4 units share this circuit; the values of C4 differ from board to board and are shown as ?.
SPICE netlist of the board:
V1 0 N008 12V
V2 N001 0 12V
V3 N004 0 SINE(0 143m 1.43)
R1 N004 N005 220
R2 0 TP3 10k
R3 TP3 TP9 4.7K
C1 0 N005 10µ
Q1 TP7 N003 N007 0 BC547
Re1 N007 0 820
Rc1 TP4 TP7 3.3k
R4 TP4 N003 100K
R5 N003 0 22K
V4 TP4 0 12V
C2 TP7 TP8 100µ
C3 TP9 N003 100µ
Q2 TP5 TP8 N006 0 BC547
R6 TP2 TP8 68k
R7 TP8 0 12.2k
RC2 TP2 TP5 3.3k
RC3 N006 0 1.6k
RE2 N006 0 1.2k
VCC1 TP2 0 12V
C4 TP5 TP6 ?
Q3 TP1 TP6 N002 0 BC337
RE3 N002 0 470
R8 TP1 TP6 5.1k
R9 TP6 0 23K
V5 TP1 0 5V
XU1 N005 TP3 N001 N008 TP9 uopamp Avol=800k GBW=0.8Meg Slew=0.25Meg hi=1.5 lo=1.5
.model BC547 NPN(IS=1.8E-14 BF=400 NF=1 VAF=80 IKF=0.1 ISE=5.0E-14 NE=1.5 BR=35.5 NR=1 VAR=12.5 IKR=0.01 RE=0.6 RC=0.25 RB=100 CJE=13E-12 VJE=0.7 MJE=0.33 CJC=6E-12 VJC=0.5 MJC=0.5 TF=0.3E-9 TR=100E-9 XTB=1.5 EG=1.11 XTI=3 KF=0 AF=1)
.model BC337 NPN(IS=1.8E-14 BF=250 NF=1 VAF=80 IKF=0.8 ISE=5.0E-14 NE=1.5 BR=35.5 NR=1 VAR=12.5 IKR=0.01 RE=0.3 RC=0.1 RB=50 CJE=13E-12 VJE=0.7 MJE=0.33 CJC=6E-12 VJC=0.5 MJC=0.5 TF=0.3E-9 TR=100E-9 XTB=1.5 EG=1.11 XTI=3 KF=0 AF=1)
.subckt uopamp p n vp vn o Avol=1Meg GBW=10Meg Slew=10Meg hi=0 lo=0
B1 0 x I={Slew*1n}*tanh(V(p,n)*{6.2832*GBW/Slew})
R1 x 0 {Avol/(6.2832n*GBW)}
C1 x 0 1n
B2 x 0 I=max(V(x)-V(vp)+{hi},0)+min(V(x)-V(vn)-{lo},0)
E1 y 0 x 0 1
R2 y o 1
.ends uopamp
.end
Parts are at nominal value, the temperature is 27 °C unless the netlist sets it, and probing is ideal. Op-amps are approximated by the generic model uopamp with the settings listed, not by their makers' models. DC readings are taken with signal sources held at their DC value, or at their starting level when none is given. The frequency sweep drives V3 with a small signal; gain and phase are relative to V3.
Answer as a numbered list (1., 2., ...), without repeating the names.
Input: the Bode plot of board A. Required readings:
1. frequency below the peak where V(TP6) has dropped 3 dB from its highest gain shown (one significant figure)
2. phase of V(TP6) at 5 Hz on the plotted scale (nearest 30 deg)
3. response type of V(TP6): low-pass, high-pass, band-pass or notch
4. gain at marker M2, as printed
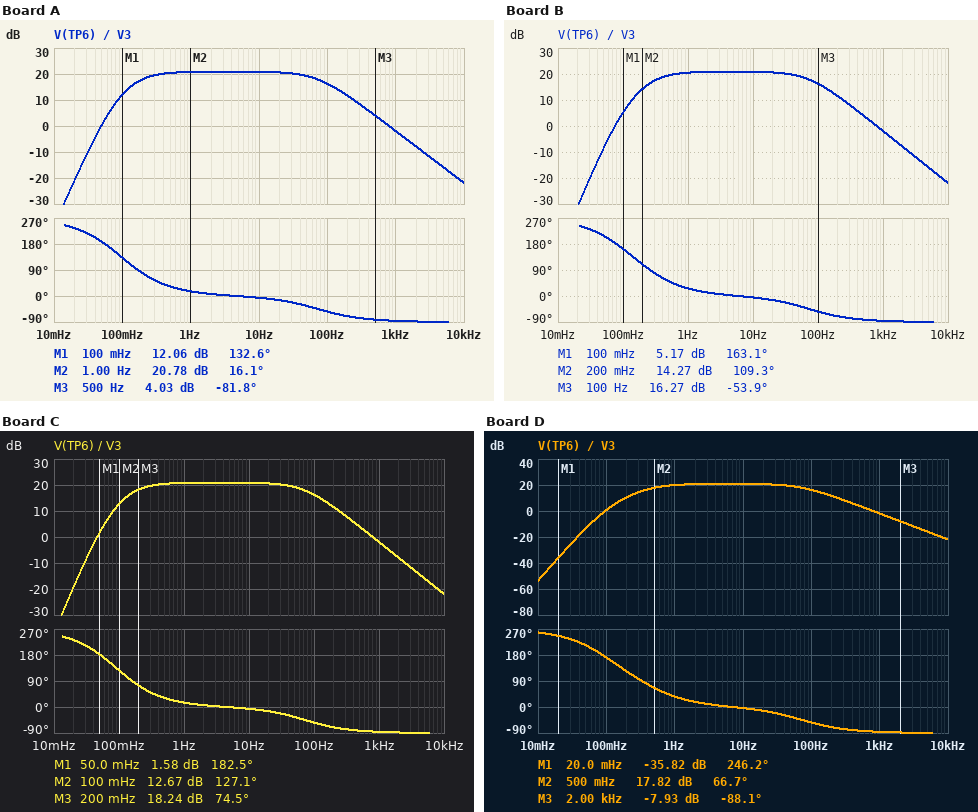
1. 200 mHz
2. 0 deg
3. band-pass
4. 20.78 dB
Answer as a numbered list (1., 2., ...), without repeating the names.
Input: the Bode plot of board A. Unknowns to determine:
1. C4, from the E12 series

1. 270 µF
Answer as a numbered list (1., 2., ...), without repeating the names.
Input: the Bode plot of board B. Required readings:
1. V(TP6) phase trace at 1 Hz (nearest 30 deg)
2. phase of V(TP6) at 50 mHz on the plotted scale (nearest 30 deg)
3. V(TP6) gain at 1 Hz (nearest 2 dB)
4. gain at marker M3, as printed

1. 30 deg
2. 210 deg
3. 20 dB
4. 16.27 dB
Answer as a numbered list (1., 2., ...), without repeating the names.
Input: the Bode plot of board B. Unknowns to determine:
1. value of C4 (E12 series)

1. 82 µF
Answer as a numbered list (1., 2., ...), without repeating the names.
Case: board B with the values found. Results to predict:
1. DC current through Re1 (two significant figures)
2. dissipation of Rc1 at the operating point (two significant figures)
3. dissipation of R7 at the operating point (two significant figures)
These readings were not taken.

1. 1.7 mA
2. 9.7 mW
3. 260 µW
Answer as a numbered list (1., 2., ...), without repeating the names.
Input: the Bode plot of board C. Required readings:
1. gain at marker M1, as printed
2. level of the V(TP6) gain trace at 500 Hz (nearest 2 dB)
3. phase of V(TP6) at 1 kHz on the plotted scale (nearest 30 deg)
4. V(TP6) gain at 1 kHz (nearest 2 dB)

1. 1.58 dB
2. 4 dB
3. -90 deg
4. -2 dB
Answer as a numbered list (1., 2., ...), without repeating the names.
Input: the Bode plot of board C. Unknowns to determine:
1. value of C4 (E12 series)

1. 330 µF
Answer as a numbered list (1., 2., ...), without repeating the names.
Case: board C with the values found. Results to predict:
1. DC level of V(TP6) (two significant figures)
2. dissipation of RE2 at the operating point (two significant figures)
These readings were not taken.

1. 4.0 V
2. 1.0 mW
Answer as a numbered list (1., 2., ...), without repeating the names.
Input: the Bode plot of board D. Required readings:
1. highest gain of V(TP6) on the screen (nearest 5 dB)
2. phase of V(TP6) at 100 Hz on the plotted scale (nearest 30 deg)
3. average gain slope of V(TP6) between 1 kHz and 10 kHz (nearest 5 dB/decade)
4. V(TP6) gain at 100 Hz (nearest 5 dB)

1. 20 dB
2. -60 deg
3. -20 dB/decade
4. 15 dB
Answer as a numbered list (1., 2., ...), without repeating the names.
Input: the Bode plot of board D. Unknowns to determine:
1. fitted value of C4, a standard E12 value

1. 47 µF
